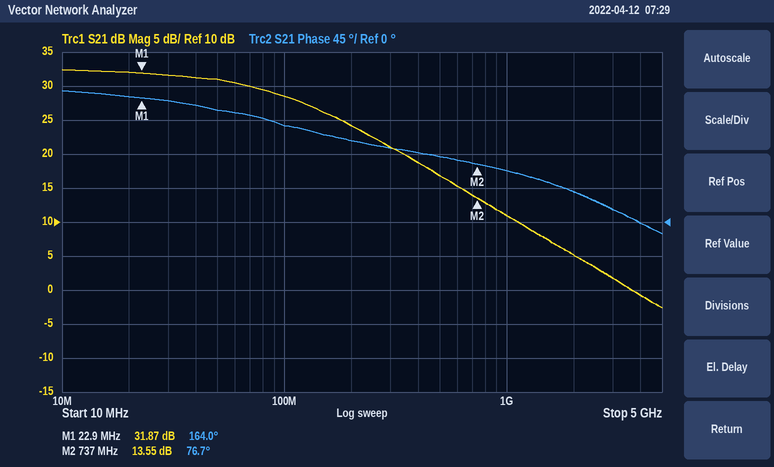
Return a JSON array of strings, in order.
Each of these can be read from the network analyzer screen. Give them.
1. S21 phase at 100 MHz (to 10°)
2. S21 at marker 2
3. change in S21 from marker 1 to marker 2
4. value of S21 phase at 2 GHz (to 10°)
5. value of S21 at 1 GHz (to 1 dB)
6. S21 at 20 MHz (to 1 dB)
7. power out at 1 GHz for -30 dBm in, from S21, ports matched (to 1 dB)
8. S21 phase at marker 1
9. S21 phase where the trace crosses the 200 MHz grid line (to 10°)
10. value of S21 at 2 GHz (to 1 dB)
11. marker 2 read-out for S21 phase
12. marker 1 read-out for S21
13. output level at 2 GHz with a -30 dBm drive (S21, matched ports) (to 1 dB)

["130°", "13.55 dB", "-18.32 dB", "40°", "11 dB", "32 dB", "-19 dBm", "164.0°", "110°", "5 dB", "76.7°", "31.87 dB", "-25 dBm"]
